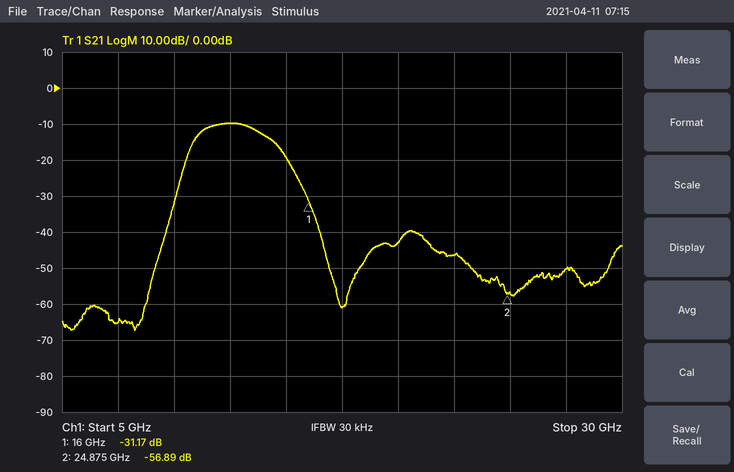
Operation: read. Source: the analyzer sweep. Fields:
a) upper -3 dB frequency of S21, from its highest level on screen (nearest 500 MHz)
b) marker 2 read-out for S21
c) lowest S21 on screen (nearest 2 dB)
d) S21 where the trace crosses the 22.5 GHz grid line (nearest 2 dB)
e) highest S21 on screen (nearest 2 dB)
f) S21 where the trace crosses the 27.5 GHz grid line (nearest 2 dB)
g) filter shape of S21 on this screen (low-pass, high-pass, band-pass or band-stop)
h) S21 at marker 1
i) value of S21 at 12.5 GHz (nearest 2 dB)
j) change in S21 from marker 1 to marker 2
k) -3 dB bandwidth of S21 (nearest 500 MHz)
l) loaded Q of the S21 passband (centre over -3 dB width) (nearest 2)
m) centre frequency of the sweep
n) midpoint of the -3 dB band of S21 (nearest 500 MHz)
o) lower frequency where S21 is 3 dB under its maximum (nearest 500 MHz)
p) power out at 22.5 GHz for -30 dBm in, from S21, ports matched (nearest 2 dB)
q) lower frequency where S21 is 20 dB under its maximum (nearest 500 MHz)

14.0 GHz
-56.89 dB
-68 dB
-46 dB
-10 dB
-50 dB
band-pass
-31.17 dB
-10 dB
-25.72 dB
3.0 GHz
4
17.5 GHz
12.5 GHz
11.0 GHz
-76 dBm
10.0 GHz
